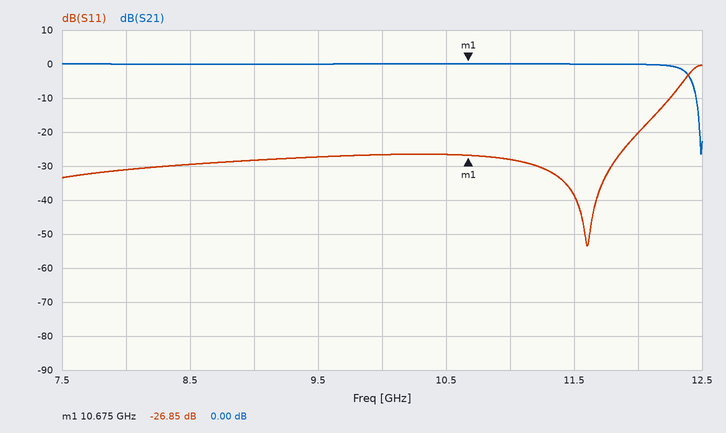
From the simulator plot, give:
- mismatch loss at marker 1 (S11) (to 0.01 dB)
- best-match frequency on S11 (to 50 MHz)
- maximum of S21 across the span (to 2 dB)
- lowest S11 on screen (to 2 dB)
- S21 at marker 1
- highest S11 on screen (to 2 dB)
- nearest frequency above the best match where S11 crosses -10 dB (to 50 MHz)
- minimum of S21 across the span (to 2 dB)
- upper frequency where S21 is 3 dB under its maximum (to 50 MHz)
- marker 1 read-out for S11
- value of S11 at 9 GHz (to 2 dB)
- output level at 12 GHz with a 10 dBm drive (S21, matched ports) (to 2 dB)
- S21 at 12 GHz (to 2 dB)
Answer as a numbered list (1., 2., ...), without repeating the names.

1. 0.01 dB
2. 11.60 GHz
3. 0 dB
4. -54 dB
5. 0.00 dB
6. 0 dB
7. 12.25 GHz
8. -26 dB
9. 12.40 GHz
10. -26.85 dB
11. -28 dB
12. 10 dBm
13. 0 dB
